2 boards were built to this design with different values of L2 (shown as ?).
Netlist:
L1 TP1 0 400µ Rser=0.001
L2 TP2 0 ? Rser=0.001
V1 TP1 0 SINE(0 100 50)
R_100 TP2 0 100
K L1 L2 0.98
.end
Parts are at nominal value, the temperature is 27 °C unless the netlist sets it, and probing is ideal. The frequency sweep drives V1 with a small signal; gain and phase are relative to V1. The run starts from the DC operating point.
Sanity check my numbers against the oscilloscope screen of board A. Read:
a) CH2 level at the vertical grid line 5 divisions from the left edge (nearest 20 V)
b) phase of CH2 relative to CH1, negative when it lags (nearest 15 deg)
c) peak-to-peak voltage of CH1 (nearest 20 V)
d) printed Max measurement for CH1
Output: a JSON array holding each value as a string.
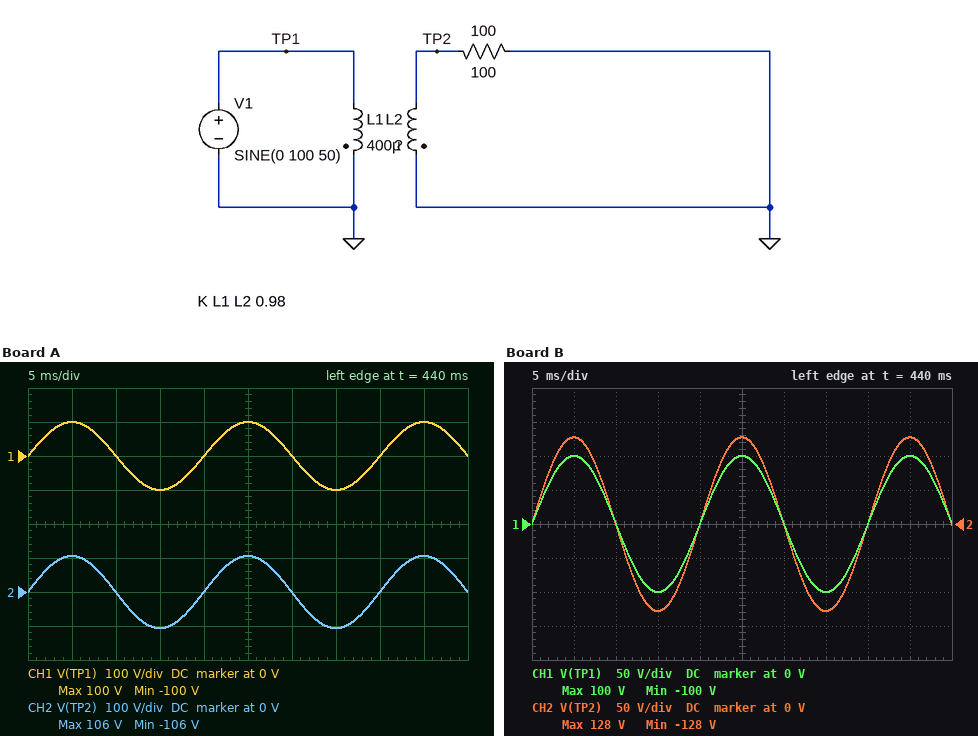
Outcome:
["100 V", "0 deg", "200 V", "100 V"]
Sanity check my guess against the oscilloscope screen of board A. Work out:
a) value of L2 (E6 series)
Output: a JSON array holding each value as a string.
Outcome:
["470 µH"]
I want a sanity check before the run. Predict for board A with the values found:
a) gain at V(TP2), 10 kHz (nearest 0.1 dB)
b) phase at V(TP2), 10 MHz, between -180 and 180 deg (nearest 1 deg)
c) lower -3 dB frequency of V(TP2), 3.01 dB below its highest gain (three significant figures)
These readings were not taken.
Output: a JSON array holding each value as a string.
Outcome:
["0.5 dB", "-85 deg", "398 mHz"]
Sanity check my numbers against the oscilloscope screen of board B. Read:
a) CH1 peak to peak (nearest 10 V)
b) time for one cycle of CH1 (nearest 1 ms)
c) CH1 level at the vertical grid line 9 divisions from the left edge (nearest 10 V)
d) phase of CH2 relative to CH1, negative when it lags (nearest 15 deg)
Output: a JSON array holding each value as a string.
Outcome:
["200 V", "20 ms", "100 V", "0 deg"]
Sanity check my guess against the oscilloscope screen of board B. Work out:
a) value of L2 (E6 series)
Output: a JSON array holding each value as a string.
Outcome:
["680 µH"]
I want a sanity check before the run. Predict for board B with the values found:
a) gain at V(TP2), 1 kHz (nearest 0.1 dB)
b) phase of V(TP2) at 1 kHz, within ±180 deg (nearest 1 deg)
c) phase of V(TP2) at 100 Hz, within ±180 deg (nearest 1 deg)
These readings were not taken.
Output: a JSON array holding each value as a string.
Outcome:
["2.1 dB", "0 deg", "0 deg"]
